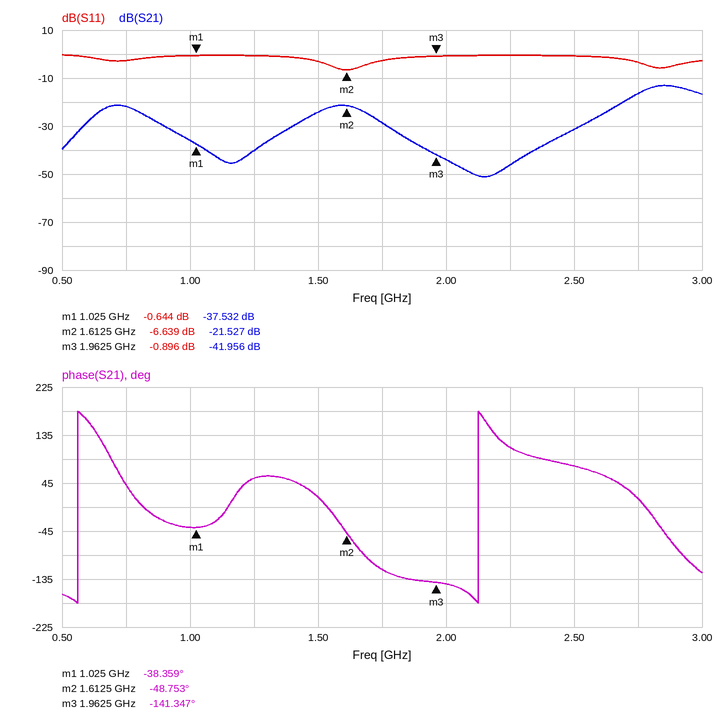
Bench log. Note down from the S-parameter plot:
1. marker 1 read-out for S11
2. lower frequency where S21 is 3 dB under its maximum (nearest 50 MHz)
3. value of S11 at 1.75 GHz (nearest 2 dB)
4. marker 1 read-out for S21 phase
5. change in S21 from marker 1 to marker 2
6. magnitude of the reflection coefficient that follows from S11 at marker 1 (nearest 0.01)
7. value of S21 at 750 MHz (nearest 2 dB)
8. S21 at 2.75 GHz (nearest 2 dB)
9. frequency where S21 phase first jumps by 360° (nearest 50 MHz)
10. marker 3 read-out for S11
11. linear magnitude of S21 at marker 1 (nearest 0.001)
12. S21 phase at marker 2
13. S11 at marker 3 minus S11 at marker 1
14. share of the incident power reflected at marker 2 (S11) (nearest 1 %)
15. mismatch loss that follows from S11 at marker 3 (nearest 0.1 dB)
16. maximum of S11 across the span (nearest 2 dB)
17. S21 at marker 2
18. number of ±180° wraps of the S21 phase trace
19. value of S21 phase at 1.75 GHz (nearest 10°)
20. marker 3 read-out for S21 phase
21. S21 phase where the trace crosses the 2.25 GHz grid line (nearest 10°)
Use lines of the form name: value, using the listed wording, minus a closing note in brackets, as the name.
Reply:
marker 1 read-out for S11: -0.644 dB
lower frequency where S21 is 3 dB under its maximum: 2.75 GHz
value of S11 at 1.75 GHz: -2 dB
marker 1 read-out for S21 phase: -38.359°
change in S21 from marker 1 to marker 2: 16.005 dB
magnitude of the reflection coefficient that follows from S11 at marker 1: 0.93
value of S21 at 750 MHz: -22 dB
S21 at 2.75 GHz: -16 dB
frequency where S21 phase first jumps by 360°: 550 MHz
marker 3 read-out for S11: -0.896 dB
linear magnitude of S21 at marker 1: 0.013
S21 phase at marker 2: -48.753°
S11 at marker 3 minus S11 at marker 1: -0.252 dB
share of the incident power reflected at marker 2 (S11): 22 %
mismatch loss that follows from S11 at marker 3: 7.3 dB
maximum of S11 across the span: 0 dB
S21 at marker 2: -21.527 dB
number of ±180° wraps of the S21 phase trace: 2
value of S21 phase at 1.75 GHz: -120°
marker 3 read-out for S21 phase: -141.347°
S21 phase where the trace crosses the 2.25 GHz grid line: 110°
